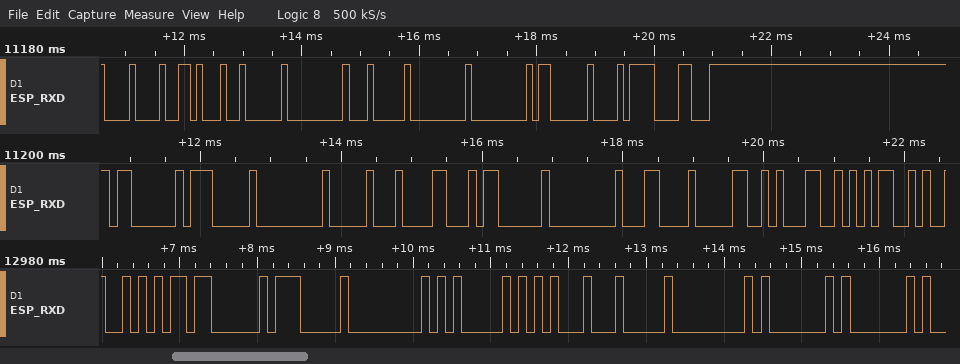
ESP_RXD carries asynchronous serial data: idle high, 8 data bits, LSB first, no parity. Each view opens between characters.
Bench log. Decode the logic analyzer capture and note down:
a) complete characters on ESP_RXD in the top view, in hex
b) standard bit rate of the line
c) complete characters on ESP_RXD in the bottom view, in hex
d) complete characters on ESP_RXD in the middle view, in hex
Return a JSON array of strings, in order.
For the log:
["08, 16, 02, 00, 04, 00, 00, 03, E8, 18", "9600 baud", "AA, 03, 07, 00, 05, 15, 04, 00, 01, 01", "03, 07, 00, 10, 18, 03, 00, 0C, 30, 31, 35"]
